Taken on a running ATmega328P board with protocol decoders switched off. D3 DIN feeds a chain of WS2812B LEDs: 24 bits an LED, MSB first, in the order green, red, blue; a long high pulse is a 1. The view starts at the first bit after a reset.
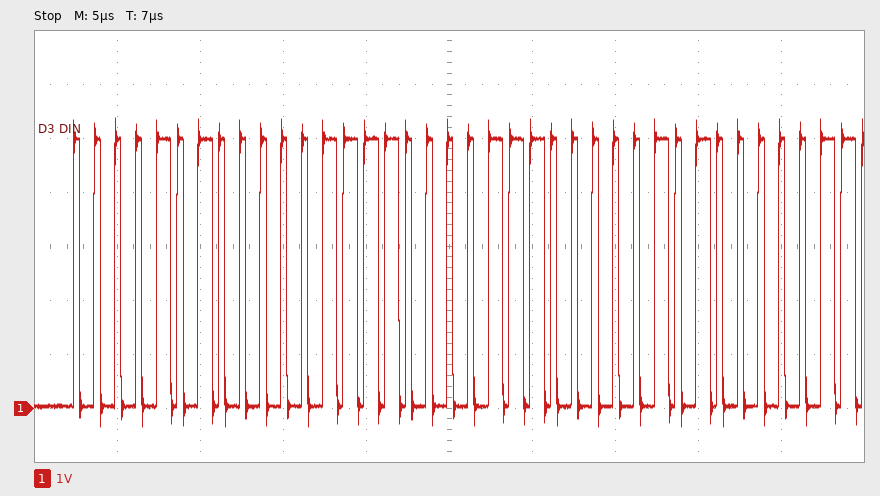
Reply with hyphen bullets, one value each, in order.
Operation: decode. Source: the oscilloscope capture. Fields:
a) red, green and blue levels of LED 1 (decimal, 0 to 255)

- 15, 10, 14
